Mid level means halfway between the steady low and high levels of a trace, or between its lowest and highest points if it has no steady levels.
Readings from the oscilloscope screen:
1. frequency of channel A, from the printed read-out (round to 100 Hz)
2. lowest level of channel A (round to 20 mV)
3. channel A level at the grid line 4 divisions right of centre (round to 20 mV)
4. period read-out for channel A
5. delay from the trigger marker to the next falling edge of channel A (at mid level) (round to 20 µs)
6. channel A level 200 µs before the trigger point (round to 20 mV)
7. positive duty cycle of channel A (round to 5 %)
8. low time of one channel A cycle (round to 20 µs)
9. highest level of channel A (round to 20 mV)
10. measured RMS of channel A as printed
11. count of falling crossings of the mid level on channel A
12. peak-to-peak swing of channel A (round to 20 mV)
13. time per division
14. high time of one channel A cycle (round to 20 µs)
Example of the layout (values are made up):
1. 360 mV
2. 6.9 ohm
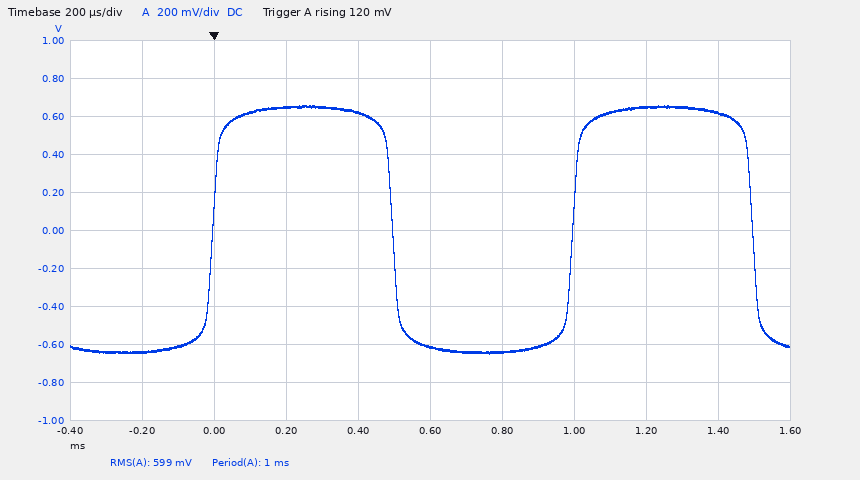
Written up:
1. 1.0 kHz
2. -640 mV
3. 620 mV
4. 1 ms
5. 500 µs
6. -640 mV
7. 50 %
8. 500 µs
9. 660 mV
10. 599 mV
11. 2
12. 1.30 V
13. 200 µs
14. 500 µs
